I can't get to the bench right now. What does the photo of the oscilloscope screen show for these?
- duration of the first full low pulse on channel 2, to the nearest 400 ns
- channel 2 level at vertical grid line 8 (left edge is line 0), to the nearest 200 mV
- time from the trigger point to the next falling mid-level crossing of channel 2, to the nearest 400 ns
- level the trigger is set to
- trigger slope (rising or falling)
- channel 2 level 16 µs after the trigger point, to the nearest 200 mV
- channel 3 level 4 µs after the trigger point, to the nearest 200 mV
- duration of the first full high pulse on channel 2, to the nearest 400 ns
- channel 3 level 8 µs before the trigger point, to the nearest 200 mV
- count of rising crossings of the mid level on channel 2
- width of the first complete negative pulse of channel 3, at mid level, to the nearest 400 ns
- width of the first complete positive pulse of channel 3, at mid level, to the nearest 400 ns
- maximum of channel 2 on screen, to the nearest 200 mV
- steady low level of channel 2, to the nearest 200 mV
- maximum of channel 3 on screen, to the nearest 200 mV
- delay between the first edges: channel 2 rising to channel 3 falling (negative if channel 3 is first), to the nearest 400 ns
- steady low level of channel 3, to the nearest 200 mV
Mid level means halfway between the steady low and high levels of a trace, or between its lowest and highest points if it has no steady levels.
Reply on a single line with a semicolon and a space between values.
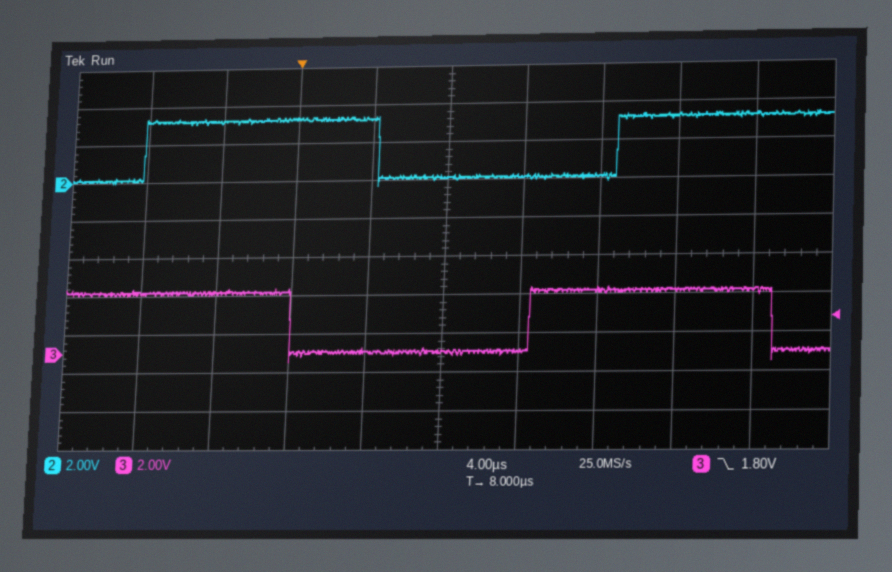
12.4 µs; 3.2 V; 4.4 µs; 1.80 V; falling; 200 mV; 200 mV; 12.4 µs; 3.2 V; 2; 12.4 µs; 12.4 µs; 3.4 V; 200 mV; 3.4 V; +8.0 µs; 0.0 V
